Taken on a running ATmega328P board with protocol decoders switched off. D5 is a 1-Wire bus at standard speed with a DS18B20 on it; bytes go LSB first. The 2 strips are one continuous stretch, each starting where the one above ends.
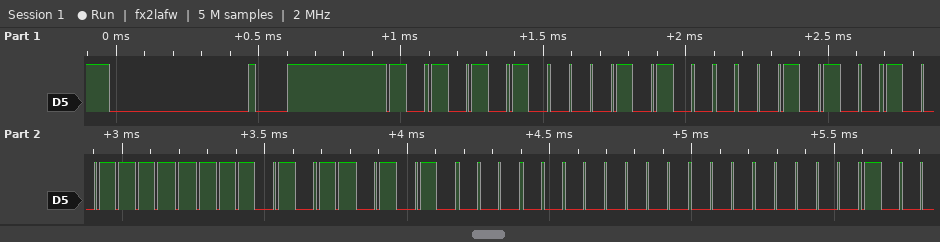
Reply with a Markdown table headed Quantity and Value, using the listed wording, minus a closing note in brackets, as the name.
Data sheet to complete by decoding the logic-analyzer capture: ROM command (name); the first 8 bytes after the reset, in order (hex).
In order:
| Quantity | Value |
|---|---|
| ROM command | Match ROM |
| the first 8 bytes after the reset, in order | 55 28 28 F9 D7 0A 00 00 |
